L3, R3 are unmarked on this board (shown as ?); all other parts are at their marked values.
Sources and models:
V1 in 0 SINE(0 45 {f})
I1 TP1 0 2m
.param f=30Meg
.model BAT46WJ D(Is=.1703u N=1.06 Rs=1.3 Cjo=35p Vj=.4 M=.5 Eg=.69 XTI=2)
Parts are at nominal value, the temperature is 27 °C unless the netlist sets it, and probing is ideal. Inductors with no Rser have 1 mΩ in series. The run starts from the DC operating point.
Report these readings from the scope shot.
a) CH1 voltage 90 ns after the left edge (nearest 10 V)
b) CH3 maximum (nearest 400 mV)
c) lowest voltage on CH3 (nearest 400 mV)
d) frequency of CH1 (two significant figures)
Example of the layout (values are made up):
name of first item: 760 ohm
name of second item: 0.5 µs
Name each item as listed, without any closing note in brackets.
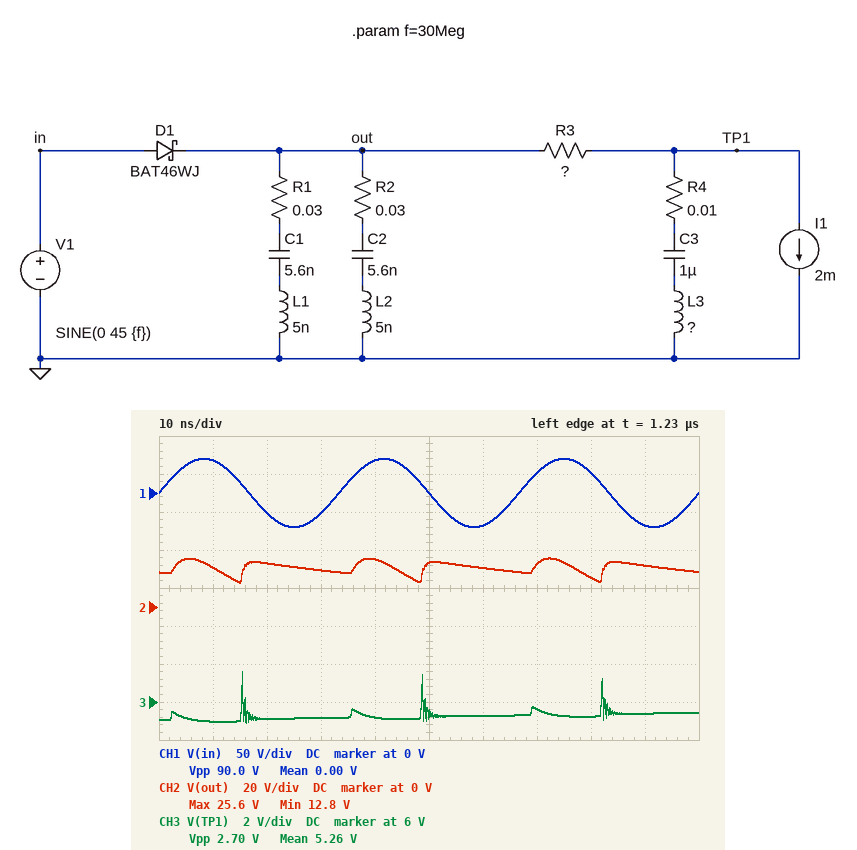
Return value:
CH1 voltage 90 ns after the left edge: -40 V
CH3 maximum: 7.6 V
lowest voltage on CH3: 4.8 V
frequency of CH1: 30 MHz
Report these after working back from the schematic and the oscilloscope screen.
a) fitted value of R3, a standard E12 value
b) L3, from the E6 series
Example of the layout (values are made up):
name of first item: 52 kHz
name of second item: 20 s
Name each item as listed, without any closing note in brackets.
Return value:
fitted value of R3, a standard E12 value: 3.9 Ω
L3, from the E6 series: 330 pH
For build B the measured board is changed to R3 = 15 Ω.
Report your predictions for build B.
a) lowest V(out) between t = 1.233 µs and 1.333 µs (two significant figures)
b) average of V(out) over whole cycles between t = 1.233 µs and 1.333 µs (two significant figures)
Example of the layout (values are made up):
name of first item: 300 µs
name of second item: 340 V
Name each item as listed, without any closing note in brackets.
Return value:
lowest V(out) between t = 1.233 µs and 1.333 µs: 22 V
average of V(out) over whole cycles between t = 1.233 µs and 1.333 µs: 30 V
